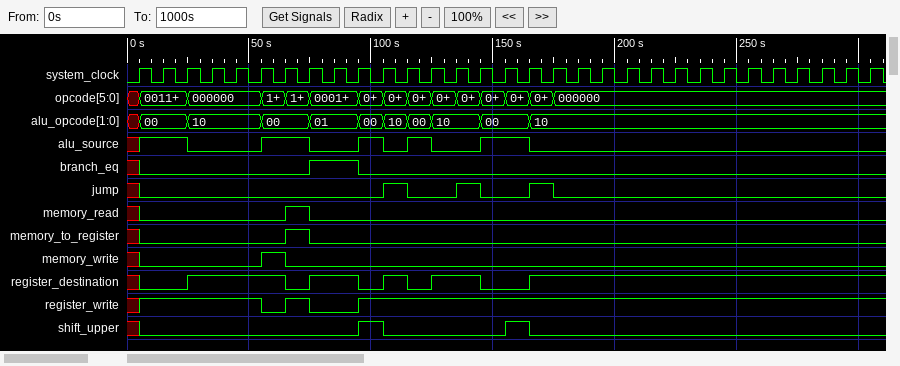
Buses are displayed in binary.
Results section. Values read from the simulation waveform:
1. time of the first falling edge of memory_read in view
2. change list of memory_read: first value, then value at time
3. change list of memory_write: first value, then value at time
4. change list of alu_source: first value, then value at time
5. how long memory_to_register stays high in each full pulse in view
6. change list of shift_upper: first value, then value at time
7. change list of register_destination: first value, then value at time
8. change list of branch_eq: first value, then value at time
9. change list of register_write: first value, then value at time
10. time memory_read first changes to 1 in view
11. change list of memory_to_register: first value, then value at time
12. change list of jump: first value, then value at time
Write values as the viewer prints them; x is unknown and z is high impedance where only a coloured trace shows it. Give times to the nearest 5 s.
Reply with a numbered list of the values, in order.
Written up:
1. 75 s
2. x, 0 at 5 s, 1 at 65 s, 0 at 75 s
3. x, 0 at 5 s, 1 at 55 s, 0 at 65 s
4. x, 1 at 5 s, 0 at 25 s, 1 at 55 s, 0 at 75 s, 1 at 95 s, 0 at 105 s, 1 at 115 s, 0 at 125 s, 1 at 145 s, 0 at 165 s
5. 10 s
6. x, 0 at 5 s, 1 at 95 s, 0 at 105 s, 1 at 155 s, 0 at 165 s
7. x, 0 at 5 s, 1 at 25 s, 0 at 65 s, 1 at 75 s, 0 at 95 s, 1 at 105 s, 0 at 115 s, 1 at 125 s, 0 at 145 s, 1 at 165 s
8. x, 0 at 5 s, 1 at 75 s, 0 at 95 s
9. x, 1 at 5 s, 0 at 55 s, 1 at 65 s, 0 at 75 s, 1 at 95 s
10. 65 s
11. x, 0 at 5 s, 1 at 65 s, 0 at 75 s
12. x, 0 at 5 s, 1 at 105 s, 0 at 115 s, 1 at 135 s, 0 at 145 s, 1 at 165 s, 0 at 175 s
